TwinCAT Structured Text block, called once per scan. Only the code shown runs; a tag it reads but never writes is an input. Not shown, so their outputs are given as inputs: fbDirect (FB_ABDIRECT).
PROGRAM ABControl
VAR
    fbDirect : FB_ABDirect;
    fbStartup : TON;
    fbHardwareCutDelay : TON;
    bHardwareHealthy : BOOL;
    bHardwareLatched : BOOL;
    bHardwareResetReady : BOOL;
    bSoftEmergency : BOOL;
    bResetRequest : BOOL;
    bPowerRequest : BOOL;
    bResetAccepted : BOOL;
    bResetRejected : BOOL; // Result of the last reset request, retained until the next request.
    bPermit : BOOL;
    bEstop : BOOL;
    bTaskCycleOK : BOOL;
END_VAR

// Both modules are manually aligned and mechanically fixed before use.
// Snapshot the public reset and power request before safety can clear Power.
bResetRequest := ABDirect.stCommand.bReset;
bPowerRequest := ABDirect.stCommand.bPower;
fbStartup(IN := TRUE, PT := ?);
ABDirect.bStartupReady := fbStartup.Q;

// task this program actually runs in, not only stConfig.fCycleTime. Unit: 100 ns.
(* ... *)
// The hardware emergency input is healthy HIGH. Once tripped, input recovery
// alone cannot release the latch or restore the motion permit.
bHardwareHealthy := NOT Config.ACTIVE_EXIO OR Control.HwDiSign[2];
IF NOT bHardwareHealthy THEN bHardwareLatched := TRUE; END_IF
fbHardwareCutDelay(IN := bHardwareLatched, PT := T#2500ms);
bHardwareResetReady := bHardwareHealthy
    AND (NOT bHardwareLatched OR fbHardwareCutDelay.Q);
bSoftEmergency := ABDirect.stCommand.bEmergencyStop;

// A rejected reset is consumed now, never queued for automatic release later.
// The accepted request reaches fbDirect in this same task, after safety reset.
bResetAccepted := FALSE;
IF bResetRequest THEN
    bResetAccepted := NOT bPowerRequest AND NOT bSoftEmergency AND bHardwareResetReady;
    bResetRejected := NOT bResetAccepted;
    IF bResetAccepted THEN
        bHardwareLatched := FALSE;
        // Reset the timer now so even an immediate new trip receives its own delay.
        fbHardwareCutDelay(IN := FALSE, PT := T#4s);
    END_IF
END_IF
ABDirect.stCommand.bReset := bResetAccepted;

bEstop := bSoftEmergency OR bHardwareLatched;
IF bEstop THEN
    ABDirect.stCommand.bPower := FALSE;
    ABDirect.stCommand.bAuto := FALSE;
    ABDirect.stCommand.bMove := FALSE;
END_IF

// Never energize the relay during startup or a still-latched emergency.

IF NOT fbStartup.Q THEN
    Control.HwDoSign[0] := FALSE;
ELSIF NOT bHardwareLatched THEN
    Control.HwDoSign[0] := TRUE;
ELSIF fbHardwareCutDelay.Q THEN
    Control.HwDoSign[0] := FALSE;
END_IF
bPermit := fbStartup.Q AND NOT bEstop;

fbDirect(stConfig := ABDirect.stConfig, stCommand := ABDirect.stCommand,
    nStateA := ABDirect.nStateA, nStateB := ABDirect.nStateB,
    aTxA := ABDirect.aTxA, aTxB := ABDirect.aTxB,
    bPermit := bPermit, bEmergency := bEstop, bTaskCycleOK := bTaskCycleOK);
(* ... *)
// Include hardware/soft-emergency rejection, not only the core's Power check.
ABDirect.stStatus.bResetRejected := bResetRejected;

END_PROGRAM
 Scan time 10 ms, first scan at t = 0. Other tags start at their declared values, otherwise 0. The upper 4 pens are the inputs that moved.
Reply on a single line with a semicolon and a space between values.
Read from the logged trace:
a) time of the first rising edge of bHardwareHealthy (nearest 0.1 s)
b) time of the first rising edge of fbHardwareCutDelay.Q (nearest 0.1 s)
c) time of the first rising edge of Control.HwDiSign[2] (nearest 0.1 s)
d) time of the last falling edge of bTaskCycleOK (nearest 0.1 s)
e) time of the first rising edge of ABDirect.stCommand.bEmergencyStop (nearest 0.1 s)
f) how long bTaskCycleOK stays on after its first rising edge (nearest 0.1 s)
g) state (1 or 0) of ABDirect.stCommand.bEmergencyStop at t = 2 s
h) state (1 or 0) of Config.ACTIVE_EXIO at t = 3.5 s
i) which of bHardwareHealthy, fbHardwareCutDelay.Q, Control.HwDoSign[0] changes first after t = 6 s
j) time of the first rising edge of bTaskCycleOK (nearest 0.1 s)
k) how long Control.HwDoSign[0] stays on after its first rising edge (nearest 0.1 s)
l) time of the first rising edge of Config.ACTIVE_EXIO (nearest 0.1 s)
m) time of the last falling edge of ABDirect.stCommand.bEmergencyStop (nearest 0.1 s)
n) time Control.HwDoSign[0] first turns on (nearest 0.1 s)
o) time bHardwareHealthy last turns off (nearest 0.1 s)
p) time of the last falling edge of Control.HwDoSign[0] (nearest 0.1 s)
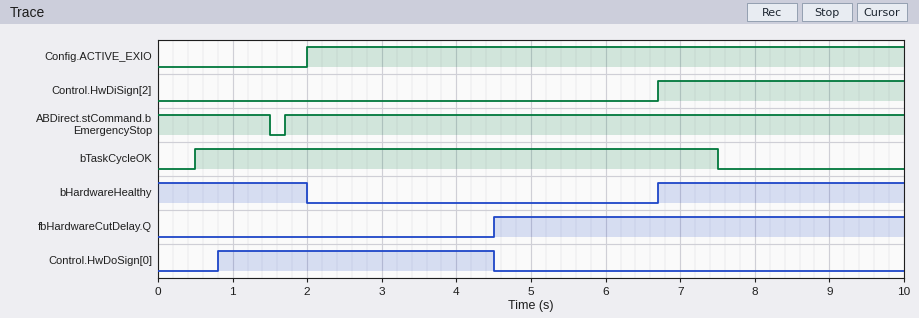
6.7 s; 4.5 s; 6.7 s; 7.5 s; 1.7 s; 7.0 s; 1; 1; bHardwareHealthy; 0.5 s; 3.7 s; 2.0 s; 1.5 s; 0.8 s; 2.0 s; 4.5 s
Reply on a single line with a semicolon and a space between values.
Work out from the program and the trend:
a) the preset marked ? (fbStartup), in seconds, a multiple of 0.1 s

0.8 s
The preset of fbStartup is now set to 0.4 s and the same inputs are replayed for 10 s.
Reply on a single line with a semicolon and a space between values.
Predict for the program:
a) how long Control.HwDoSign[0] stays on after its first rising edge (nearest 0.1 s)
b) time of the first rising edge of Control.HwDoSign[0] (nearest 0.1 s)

4.1 s; 0.4 s
